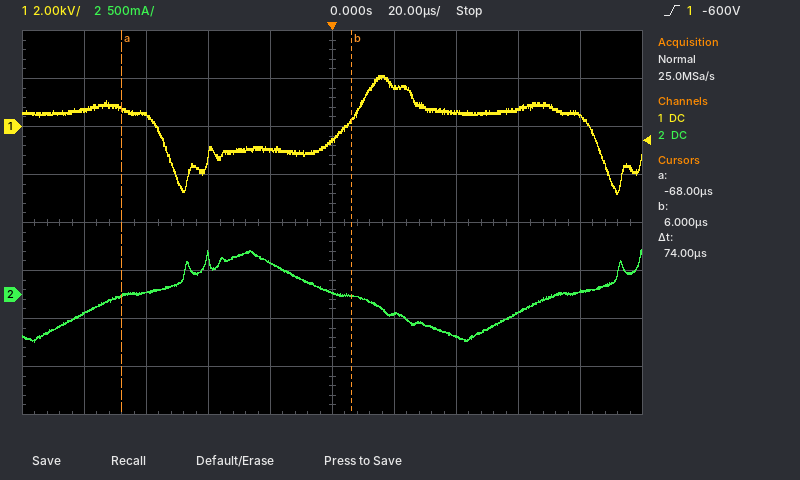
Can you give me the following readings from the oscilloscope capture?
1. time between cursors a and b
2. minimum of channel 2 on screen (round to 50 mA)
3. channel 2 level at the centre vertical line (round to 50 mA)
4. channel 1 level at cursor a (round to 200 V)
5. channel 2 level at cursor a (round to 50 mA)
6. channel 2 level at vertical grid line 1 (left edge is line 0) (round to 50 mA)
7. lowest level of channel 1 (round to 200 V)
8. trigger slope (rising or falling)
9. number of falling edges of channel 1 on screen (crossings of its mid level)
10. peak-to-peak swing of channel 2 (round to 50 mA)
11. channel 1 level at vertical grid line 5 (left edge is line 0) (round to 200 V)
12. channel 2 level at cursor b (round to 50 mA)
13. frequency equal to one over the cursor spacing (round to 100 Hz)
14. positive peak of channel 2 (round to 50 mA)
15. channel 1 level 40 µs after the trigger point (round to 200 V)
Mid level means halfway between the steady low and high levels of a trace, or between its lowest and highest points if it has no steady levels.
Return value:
74 µs
-500 mA
0 mA
800 V
0 mA
-200 mA
-2.8 kV
rising
2
950 mA
-600 V
0 mA
13.5 kHz
450 mA
600 V
